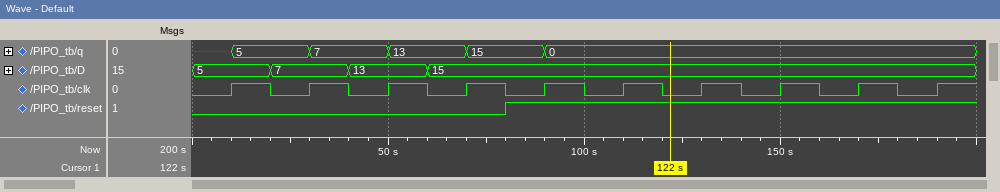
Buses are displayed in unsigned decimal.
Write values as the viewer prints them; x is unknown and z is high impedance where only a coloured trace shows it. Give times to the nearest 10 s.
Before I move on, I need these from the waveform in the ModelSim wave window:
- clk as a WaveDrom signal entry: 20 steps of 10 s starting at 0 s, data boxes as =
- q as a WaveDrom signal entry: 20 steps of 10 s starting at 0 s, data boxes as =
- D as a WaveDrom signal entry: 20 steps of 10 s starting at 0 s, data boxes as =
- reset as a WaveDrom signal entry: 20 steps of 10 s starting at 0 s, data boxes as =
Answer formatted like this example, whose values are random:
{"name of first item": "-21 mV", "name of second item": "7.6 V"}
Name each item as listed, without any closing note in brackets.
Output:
{"clk as a WaveDrom signal entry: 20 steps of 10 s starting at 0 s, data boxes as =": "{name: 'clk', wave: '01010101010101010101'}", "q as a WaveDrom signal entry: 20 steps of 10 s starting at 0 s, data boxes as =": "{name: 'q', wave: 'x=.=.=.=.=..........', data: '5 7 13 15 0'}", "D as a WaveDrom signal entry: 20 steps of 10 s starting at 0 s, data boxes as =": "{name: 'D', wave: '=.=.=.=.............', data: '5 7 13 15'}", "reset as a WaveDrom signal entry: 20 steps of 10 s starting at 0 s, data boxes as =": "{name: 'reset', wave: '0.......1...........'}"}
